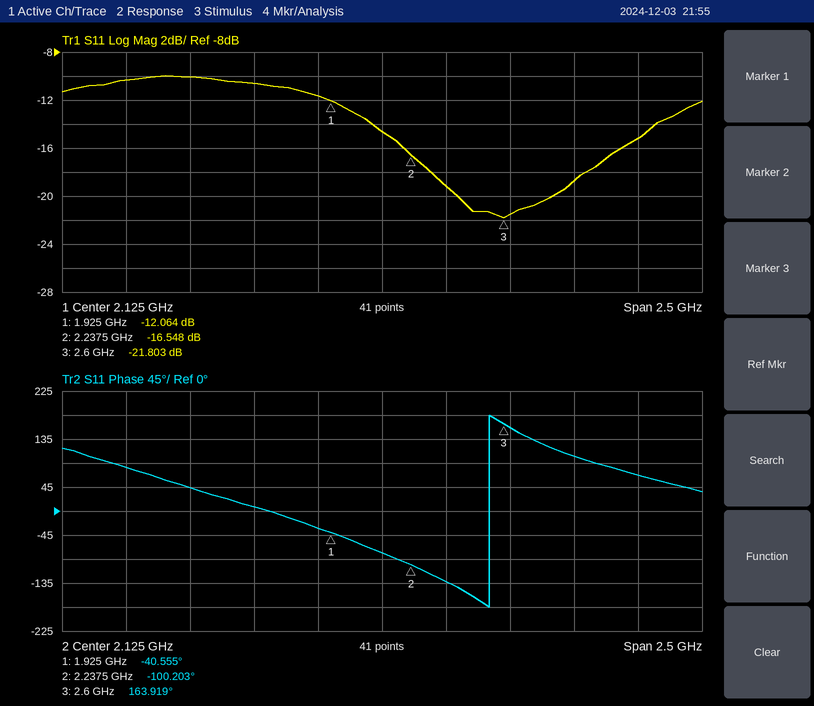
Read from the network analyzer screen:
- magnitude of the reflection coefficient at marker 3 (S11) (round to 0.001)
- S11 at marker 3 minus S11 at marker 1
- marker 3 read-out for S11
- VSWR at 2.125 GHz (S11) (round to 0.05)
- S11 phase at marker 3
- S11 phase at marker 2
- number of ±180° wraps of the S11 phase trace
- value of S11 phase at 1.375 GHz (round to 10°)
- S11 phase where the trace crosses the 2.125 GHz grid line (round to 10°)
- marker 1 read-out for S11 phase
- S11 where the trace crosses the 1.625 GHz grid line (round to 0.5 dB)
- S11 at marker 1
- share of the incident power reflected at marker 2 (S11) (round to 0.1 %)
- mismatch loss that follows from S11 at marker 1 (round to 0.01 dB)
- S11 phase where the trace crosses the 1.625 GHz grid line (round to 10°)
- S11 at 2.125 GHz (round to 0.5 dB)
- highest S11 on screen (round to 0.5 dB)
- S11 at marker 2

0.081
-9.739 dB
-21.803 dB
1.45
163.919°
-100.203°
1
40°
-80°
-40.555°
-10.5 dB
-12.064 dB
2.2 %
0.28 dB
10°
-14.5 dB
-10.0 dB
-16.548 dB
